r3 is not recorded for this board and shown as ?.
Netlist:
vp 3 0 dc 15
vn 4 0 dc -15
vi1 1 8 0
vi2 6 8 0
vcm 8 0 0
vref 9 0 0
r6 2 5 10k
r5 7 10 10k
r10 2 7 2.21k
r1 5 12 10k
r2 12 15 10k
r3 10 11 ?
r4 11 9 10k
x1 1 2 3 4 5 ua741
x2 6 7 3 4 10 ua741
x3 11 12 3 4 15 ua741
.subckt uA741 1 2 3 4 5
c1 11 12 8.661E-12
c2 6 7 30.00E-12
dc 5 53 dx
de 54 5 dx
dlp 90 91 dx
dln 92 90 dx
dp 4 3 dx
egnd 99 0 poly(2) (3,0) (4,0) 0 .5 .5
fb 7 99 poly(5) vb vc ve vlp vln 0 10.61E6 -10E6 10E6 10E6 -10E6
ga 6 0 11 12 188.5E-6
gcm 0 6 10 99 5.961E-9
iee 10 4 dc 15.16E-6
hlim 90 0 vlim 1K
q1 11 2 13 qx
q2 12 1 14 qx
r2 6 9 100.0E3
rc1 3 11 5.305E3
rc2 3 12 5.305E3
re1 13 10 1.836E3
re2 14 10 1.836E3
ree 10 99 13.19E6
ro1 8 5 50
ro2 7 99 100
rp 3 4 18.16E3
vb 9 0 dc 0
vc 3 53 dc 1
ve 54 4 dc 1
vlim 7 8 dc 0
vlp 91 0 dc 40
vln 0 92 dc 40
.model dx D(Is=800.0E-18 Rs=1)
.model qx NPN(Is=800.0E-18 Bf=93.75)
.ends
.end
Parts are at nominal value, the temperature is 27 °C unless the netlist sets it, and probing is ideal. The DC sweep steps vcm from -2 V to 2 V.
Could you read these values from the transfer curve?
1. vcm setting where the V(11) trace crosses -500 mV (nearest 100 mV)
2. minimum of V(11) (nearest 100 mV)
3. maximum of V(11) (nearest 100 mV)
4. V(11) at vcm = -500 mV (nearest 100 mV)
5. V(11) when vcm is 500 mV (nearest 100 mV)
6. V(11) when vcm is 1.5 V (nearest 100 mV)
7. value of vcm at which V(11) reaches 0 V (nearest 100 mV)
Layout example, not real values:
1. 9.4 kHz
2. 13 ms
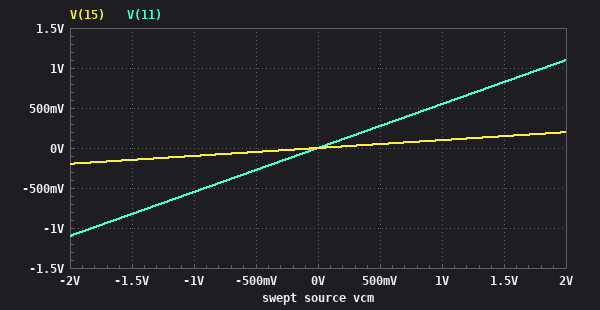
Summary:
1. -900 mV
2. -1.1 V
3. 1.1 V
4. -300 mV
5. 300 mV
6. 800 mV
7. 0 V
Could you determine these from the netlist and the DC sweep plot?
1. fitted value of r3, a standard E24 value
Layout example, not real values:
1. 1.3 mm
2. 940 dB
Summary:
1. 8.2 kΩ
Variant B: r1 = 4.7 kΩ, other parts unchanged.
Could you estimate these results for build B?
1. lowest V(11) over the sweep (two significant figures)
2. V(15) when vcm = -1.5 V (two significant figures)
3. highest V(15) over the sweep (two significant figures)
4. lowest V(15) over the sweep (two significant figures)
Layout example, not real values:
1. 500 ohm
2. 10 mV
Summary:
1. -1.1 V
2. 610 mV
3. 820 mV
4. -820 mV
